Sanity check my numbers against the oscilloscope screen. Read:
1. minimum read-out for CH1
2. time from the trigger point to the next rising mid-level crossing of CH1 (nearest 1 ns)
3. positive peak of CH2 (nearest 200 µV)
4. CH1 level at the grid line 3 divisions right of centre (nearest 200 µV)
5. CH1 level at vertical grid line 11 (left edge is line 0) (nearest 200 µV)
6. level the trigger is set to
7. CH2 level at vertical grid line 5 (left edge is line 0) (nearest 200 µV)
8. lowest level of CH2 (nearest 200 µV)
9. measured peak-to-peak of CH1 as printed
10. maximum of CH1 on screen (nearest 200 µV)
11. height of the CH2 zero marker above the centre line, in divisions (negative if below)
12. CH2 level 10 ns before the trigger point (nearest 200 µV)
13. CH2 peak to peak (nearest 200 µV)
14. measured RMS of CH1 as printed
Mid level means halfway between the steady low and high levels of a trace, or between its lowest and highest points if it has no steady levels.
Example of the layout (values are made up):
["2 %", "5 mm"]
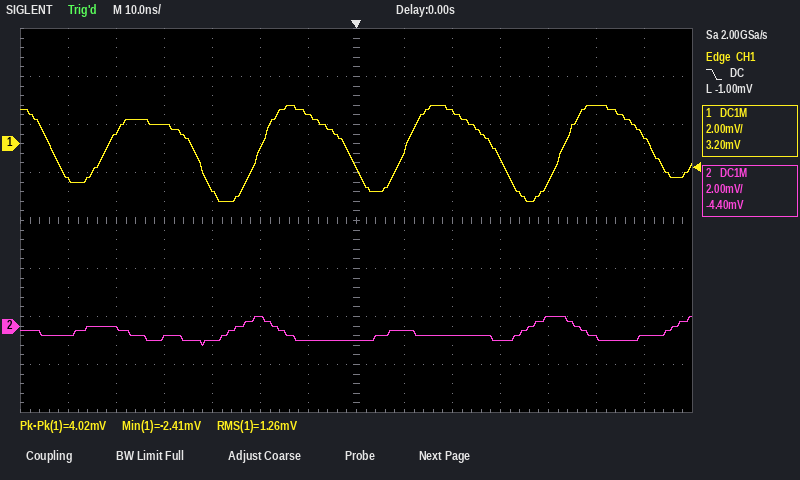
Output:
["-2.41 mV", "10 ns", "400 µV", "-600 µV", "-1.6 mV", "-1.00 mV", "400 µV", "-800 µV", "4.02 mV", "1.6 mV", "-2.2 div", "-600 µV", "1.2 mV", "1.26 mV"]
